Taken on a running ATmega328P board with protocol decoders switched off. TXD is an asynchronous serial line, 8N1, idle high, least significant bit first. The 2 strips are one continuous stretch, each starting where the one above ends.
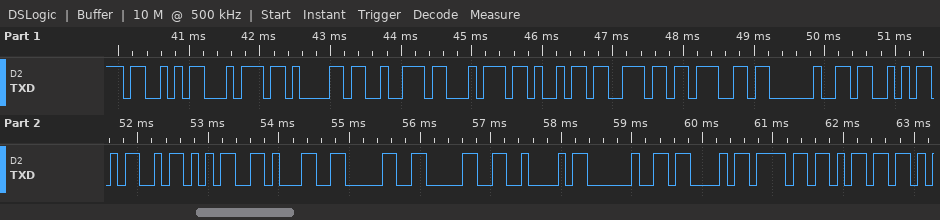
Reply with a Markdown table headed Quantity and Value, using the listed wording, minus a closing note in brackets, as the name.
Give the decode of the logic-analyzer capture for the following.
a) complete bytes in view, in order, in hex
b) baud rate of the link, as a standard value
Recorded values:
| Quantity | Value |
|---|---|
| complete bytes in view, in order, in hex | 53 74 61 72 74 69 6E 67 20 53 4D 35 31 30 30 42 20 43 6F 6D |
| baud rate of the link, as a standard value | 9600 baud |
